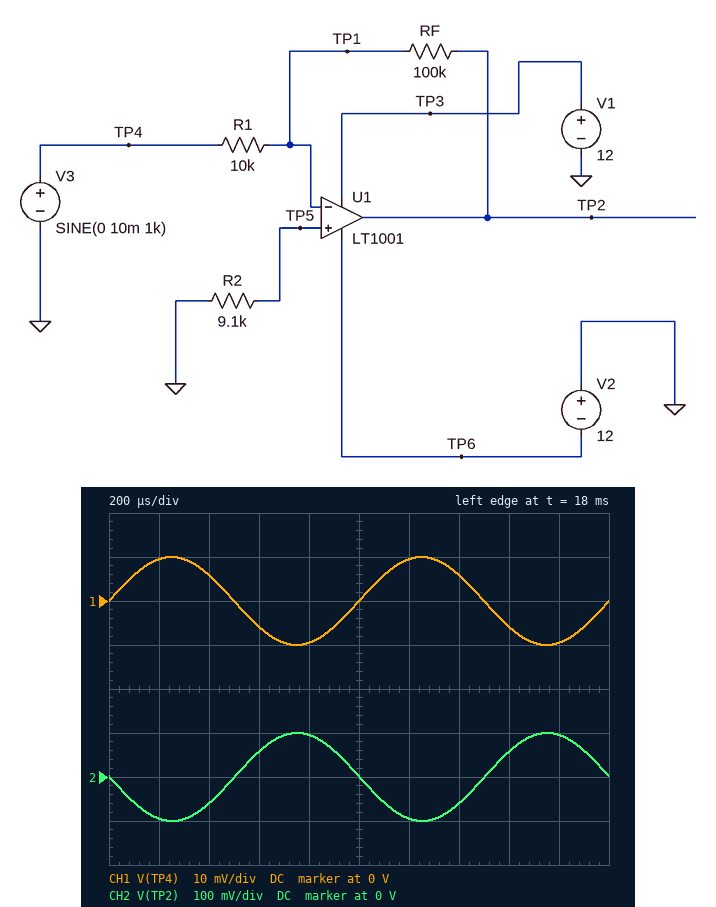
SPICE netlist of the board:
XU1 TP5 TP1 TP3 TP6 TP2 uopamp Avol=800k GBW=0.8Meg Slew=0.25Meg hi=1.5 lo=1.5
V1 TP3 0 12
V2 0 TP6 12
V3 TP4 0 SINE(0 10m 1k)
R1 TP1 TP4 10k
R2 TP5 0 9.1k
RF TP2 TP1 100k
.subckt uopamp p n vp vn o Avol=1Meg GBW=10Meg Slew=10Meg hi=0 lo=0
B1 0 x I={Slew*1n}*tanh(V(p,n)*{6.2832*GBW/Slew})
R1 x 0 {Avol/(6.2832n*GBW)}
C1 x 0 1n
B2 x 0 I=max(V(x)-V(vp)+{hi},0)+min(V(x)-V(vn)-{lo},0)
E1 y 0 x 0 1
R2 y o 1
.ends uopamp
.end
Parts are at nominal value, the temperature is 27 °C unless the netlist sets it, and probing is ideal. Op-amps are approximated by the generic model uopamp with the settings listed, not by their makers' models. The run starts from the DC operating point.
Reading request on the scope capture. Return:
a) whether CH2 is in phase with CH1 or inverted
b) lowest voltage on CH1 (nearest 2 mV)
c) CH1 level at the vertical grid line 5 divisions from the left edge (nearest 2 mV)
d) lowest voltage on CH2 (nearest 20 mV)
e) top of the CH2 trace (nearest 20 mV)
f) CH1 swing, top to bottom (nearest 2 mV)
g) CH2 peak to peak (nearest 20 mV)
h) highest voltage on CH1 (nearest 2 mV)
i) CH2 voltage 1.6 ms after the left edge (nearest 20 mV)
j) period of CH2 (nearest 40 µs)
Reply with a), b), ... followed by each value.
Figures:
a) inverted
b) -10 mV
c) 0 V
d) -100 mV
e) 100 mV
f) 20 mV
g) 200 mV
h) 10 mV
i) 60 mV
j) 1.00 ms
